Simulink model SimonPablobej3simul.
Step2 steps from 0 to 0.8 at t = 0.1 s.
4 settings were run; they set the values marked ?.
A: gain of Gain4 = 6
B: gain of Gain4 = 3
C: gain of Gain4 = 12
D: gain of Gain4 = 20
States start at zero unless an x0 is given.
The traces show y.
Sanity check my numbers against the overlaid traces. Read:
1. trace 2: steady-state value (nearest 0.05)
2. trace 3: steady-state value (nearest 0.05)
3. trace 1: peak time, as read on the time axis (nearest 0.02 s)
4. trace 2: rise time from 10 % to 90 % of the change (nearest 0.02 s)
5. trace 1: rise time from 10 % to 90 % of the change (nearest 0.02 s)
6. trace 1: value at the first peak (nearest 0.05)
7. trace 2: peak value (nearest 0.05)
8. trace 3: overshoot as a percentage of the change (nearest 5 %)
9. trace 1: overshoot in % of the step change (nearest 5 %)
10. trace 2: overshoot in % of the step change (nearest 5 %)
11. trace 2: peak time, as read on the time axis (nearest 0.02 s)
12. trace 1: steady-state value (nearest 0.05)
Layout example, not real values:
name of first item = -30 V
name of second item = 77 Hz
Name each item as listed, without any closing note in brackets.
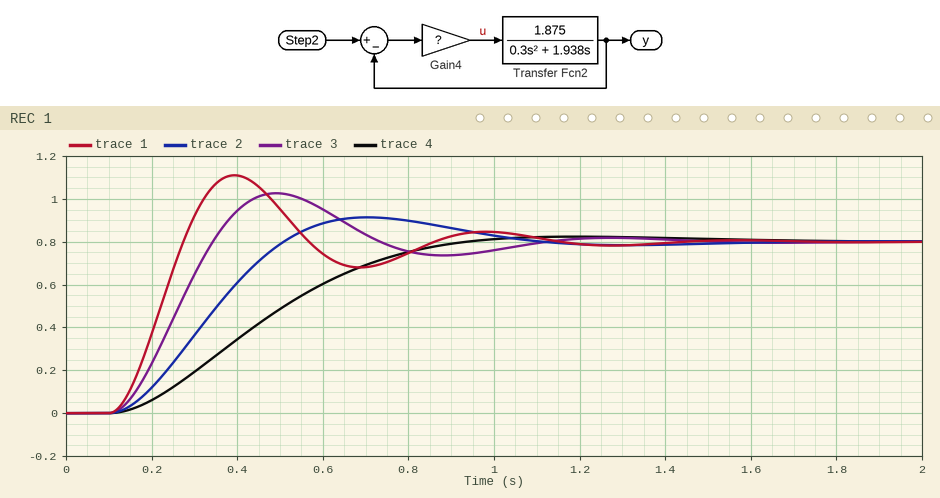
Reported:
trace 2: steady-state value = 0.80
trace 3: steady-state value = 0.80
trace 1: peak time, as read on the time axis = 0.40 s
trace 2: rise time from 10 % to 90 % of the change = 0.28 s
trace 1: rise time from 10 % to 90 % of the change = 0.12 s
trace 1: value at the first peak = 1.10
trace 2: peak value = 0.90
trace 3: overshoot as a percentage of the change = 30 %
trace 1: overshoot in % of the step change = 40 %
trace 2: overshoot in % of the step change = 15 %
trace 2: peak time, as read on the time axis = 0.70 s
trace 1: steady-state value = 0.80
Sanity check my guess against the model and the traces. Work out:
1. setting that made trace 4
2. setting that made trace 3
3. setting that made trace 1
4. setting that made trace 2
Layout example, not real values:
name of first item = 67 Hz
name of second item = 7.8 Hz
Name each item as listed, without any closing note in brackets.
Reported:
setting that made trace 4 = B
setting that made trace 3 = C
setting that made trace 1 = D
setting that made trace 2 = A
